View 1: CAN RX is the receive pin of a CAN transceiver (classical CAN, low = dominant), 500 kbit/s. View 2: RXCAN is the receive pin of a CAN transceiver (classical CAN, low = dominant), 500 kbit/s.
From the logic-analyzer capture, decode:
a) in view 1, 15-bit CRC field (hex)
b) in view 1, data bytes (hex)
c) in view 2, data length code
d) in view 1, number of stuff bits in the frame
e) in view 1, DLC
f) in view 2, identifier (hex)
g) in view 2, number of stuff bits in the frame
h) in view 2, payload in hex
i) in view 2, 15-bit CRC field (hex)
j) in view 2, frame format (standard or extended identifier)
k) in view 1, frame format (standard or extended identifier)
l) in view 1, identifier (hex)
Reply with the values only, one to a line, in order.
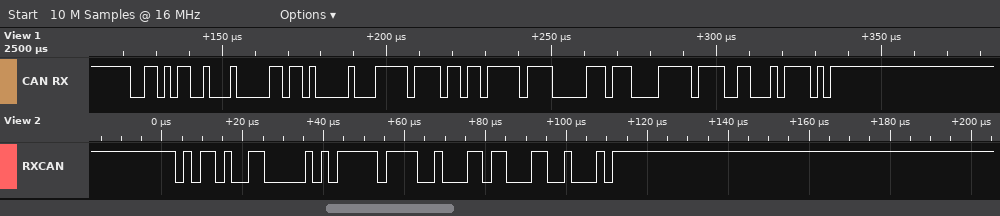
0x4C5E
2D 00 FF B6 FF 83 70 FF
2
6
8
0x5A6
2
FF 91
0x58C8
standard
standard
0x359
